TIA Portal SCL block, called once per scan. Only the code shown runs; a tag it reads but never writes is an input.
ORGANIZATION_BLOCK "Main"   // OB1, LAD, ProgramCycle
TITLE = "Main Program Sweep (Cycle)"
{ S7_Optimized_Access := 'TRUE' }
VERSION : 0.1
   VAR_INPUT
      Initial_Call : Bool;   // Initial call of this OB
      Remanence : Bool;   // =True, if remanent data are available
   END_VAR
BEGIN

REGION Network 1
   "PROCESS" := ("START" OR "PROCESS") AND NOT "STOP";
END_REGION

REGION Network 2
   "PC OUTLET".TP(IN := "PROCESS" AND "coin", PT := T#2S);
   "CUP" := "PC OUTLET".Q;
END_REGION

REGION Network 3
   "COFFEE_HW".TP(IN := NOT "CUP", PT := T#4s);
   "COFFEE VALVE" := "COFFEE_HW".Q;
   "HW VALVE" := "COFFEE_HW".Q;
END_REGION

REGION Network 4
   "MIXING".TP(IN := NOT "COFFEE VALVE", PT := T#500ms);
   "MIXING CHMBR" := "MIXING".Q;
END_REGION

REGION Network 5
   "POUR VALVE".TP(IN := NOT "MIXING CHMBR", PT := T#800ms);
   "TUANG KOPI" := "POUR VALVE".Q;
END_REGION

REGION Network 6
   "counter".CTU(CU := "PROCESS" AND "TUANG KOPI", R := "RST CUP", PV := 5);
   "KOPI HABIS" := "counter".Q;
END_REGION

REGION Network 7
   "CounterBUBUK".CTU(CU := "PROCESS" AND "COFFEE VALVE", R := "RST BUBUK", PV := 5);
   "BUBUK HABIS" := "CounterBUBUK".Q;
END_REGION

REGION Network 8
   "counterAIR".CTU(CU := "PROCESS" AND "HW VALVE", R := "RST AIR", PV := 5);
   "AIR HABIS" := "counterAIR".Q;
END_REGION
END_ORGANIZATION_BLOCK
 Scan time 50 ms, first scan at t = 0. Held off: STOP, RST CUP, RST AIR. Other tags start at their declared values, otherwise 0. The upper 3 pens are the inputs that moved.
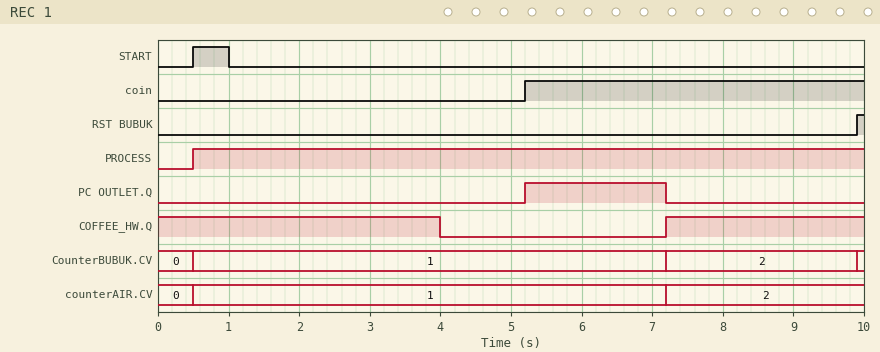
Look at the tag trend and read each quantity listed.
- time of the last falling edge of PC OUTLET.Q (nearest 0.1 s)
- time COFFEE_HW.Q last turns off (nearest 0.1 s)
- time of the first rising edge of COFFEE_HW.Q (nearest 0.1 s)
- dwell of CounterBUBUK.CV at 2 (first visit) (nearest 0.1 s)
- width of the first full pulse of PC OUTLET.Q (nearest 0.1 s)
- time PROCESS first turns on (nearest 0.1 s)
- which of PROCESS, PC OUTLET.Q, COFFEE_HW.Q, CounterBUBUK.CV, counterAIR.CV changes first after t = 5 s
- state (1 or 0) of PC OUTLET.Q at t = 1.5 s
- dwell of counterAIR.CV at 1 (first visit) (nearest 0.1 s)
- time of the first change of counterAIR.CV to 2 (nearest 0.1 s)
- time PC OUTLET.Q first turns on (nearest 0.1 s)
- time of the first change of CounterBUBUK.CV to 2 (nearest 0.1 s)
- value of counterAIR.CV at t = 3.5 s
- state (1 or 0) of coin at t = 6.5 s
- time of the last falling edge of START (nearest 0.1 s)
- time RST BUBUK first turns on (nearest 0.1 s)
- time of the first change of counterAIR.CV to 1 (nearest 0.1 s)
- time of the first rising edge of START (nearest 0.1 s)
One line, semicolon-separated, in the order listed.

7.2 s; 4.0 s; 7.2 s; 2.7 s; 2.0 s; 0.5 s; PC OUTLET.Q; 0; 6.7 s; 7.2 s; 5.2 s; 7.2 s; 1; 1; 1.0 s; 9.9 s; 0.5 s; 0.5 s
